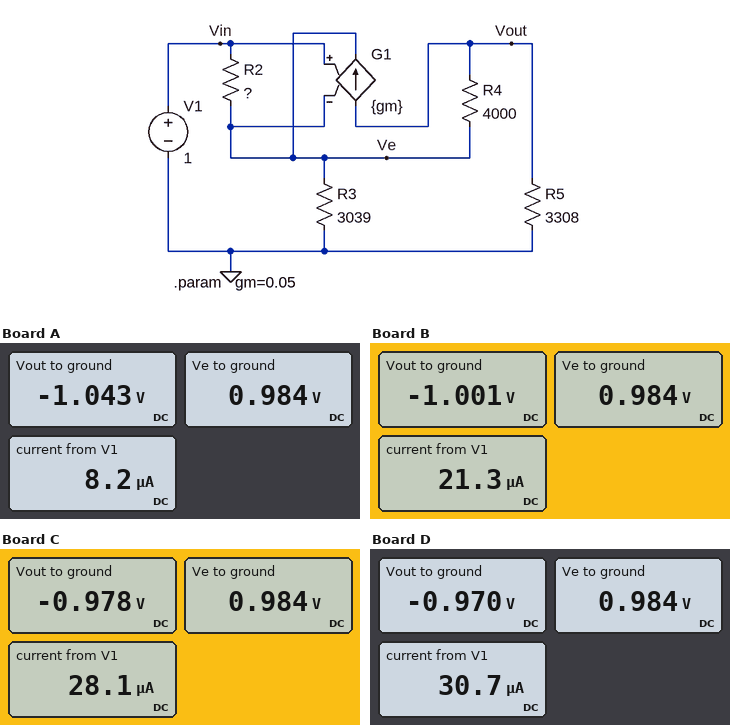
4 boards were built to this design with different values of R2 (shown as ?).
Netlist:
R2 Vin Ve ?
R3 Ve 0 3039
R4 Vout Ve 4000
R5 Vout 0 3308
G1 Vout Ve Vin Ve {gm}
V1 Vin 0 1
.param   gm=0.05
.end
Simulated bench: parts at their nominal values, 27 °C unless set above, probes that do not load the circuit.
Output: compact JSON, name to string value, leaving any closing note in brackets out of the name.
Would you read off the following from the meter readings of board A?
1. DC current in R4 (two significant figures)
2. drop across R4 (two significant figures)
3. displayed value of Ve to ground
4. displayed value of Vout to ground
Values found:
{"DC current in R4": "510 µA", "drop across R4": "2.0 V", "displayed value of Ve to ground": "0.984 V", "displayed value of Vout to ground": "-1.043 V"}
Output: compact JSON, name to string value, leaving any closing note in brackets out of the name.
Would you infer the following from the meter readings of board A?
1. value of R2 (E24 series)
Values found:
{"value of R2": "2 kΩ"}
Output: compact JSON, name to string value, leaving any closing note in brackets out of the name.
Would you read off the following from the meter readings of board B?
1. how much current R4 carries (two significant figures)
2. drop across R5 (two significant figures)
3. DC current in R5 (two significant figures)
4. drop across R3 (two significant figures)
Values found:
{"how much current R4 carries": "500 µA", "drop across R5": "1.0 V", "DC current in R5": "300 µA", "drop across R3": "980 mV"}
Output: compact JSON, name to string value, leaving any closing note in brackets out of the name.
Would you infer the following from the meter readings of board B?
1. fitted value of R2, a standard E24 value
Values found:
{"fitted value of R2, a standard E24 value": "750 Ω"}
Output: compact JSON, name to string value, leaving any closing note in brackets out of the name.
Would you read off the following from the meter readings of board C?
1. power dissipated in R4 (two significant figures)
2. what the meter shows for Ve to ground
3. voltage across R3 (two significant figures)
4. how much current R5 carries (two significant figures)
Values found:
{"power dissipated in R4": "960 µW", "what the meter shows for Ve to ground": "0.984 V", "voltage across R3": "980 mV", "how much current R5 carries": "300 µA"}
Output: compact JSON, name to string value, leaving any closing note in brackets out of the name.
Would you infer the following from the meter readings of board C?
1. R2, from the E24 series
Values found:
{"R2, from the E24 series": "560 Ω"}
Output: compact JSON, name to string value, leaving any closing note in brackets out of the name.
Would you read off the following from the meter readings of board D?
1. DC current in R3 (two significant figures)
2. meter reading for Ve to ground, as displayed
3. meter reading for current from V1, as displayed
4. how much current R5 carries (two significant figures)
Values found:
{"DC current in R3": "320 µA", "meter reading for Ve to ground, as displayed": "0.984 V", "meter reading for current from V1, as displayed": "30.7 µA", "how much current R5 carries": "290 µA"}
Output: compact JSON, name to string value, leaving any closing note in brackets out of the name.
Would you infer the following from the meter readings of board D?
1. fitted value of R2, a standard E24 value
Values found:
{"fitted value of R2, a standard E24 value": "510 Ω"}
